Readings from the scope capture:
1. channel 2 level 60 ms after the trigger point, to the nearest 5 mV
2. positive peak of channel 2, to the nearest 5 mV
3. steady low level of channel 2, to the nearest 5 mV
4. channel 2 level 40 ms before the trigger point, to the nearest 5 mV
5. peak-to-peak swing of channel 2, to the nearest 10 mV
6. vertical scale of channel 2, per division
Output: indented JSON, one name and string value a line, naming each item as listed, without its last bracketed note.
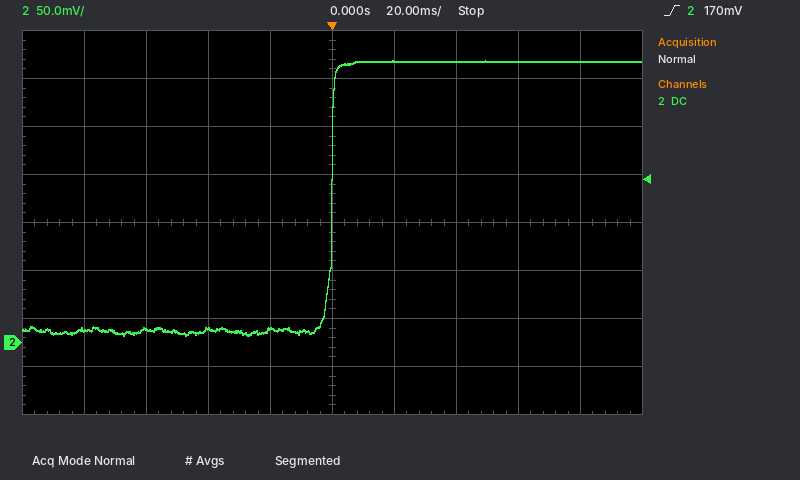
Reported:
{
  "channel 2 level 60 ms after the trigger point, to the nearest 5 mV": "295 mV",
  "positive peak of channel 2, to the nearest 5 mV": "295 mV",
  "steady low level of channel 2, to the nearest 5 mV": "10 mV",
  "channel 2 level 40 ms before the trigger point, to the nearest 5 mV": "15 mV",
  "peak-to-peak swing of channel 2, to the nearest 10 mV": "290 mV",
  "vertical scale of channel 2, per division": "50 mV"
}
